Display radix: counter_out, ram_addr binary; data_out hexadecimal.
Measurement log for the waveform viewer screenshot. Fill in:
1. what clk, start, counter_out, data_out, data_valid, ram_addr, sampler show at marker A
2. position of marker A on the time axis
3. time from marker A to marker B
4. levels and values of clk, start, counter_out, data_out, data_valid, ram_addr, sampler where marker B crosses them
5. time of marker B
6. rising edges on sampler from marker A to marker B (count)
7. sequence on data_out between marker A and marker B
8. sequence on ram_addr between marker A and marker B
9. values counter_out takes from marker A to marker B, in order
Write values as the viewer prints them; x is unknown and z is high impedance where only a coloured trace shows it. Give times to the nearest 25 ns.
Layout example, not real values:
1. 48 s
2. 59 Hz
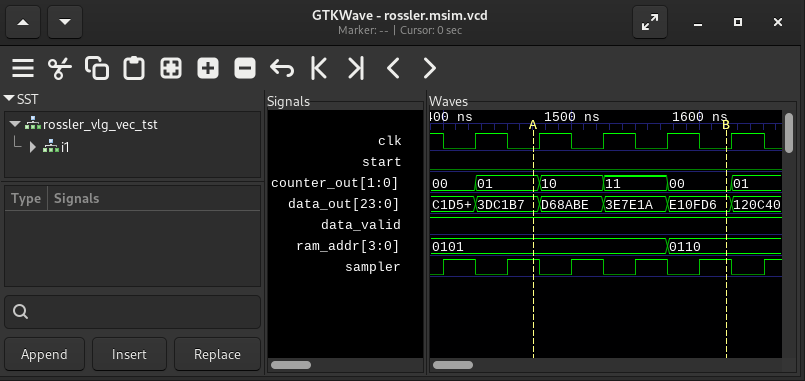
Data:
1. clk=0, start=0, counter_out=01, data_out=3DC1B7, data_valid=1, ram_addr=0101, sampler=1
2. 1475 ns
3. 150 ns
4. clk=0, start=0, counter_out=00, data_out=E10FD6, data_valid=1, ram_addr=0110, sampler=1
5. 1625 ns
6. 3
7. 3DC1B7, D68ABE, 3E7E1A, E10FD6
8. 0101, 0110
9. 01, 10, 11, 00
